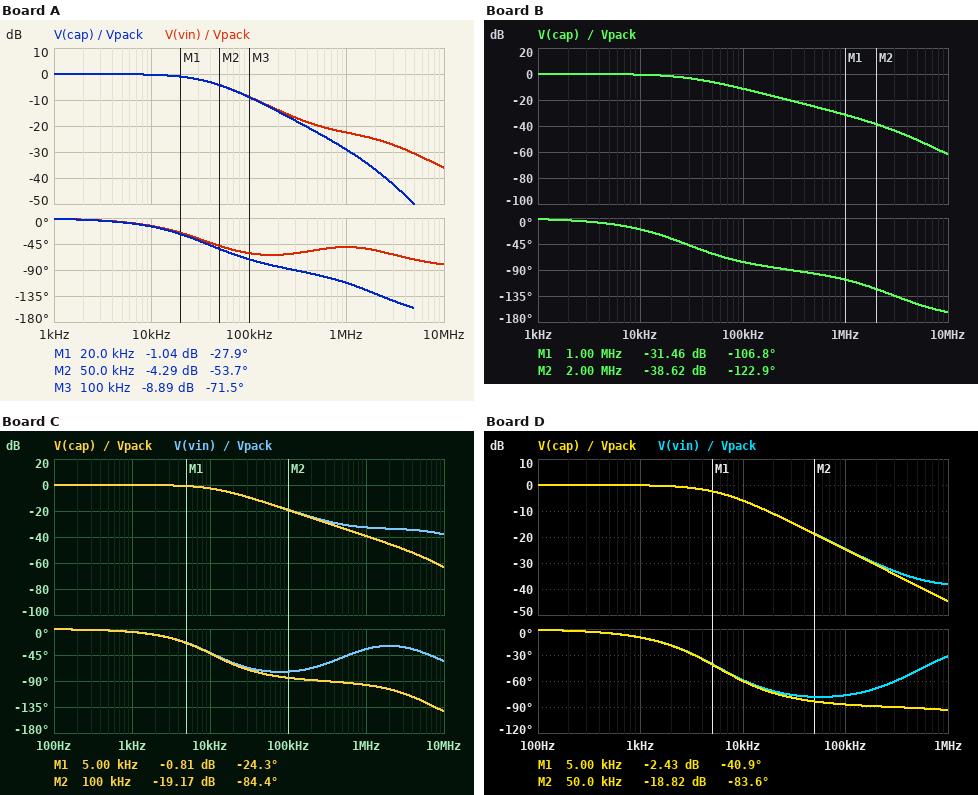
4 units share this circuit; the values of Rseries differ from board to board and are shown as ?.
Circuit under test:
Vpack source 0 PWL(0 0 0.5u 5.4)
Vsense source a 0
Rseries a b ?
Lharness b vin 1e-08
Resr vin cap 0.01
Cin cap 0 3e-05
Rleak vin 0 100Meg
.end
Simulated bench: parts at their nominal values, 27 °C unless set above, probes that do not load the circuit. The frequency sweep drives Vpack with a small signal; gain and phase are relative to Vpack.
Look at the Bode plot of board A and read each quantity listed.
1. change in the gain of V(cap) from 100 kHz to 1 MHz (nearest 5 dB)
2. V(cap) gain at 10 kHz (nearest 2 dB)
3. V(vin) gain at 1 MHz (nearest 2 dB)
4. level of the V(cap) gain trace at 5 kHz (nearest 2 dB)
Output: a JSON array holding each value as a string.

["-20 dB", "0 dB", "-22 dB", "0 dB"]
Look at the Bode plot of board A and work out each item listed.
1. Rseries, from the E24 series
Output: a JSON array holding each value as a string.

["0.13 Ω"]
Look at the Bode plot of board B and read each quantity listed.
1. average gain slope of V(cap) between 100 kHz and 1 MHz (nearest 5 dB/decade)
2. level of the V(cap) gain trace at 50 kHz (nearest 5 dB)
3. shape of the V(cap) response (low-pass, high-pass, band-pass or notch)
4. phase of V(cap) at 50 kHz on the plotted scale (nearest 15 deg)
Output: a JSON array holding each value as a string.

["-20 dB/decade", "-5 dB", "low-pass", "-60 deg"]
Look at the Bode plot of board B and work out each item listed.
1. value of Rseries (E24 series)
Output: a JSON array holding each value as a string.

["0.18 Ω"]
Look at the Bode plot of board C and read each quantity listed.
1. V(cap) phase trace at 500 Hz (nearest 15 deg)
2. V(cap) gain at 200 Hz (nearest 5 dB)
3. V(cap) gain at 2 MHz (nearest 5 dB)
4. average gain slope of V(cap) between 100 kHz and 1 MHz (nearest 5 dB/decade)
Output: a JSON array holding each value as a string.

["0 deg", "0 dB", "-45 dB", "-20 dB/decade"]
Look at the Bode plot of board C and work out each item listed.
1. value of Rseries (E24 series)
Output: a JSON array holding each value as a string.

["0.47 Ω"]
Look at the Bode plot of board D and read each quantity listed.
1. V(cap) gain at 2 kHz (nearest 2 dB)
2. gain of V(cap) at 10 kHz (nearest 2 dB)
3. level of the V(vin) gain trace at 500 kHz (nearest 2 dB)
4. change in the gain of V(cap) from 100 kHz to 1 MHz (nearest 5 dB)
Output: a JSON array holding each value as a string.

["0 dB", "-6 dB", "-36 dB", "-20 dB"]
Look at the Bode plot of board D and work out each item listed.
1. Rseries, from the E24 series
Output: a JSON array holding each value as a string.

["0.91 Ω"]
